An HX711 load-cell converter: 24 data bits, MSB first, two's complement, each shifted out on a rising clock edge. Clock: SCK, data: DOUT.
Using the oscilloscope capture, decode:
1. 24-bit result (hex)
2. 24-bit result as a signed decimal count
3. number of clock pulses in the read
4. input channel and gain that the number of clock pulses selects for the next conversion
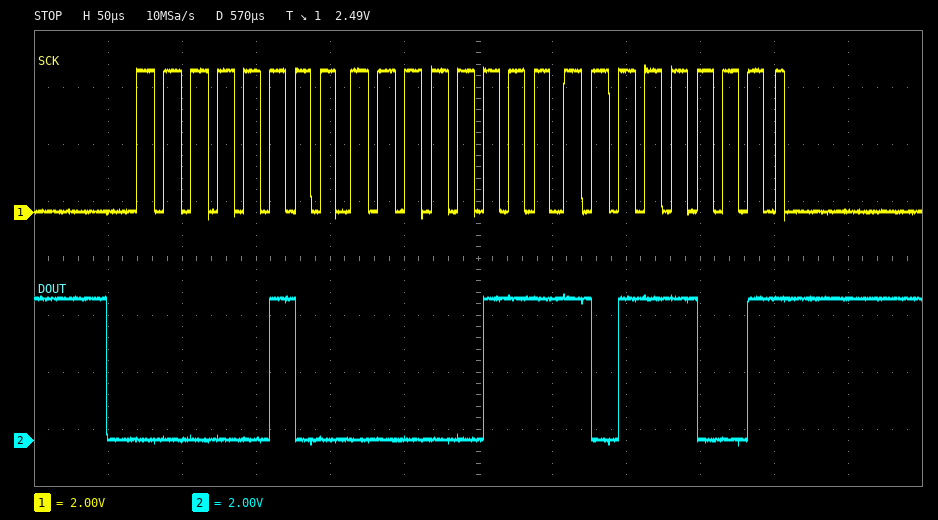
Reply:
0x0407B9
264121
25
channel A, gain 128
